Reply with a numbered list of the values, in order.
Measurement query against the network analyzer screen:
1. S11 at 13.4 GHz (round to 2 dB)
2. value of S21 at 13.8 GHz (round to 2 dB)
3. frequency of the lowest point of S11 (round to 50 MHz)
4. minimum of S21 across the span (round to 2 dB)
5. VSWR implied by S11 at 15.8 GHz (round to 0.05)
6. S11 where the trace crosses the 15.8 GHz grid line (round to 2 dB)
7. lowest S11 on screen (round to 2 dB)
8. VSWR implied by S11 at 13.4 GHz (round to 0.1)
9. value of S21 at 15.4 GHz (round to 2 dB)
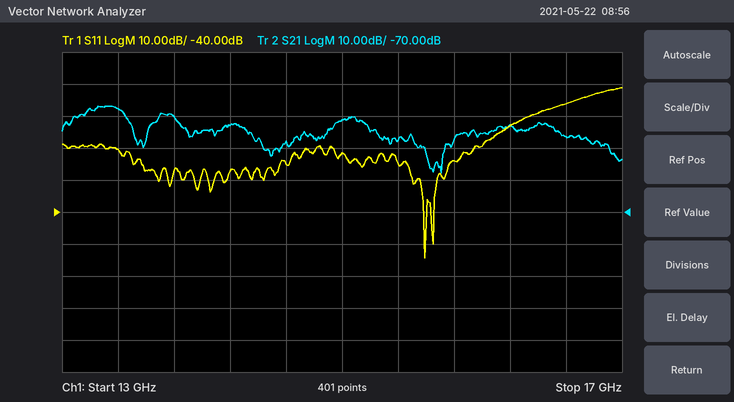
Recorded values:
1. -20 dB
2. -40 dB
3. 15.60 GHz
4. -58 dB
5. 1.15
6. -24 dB
7. -54 dB
8. 1.2
9. -48 dB
